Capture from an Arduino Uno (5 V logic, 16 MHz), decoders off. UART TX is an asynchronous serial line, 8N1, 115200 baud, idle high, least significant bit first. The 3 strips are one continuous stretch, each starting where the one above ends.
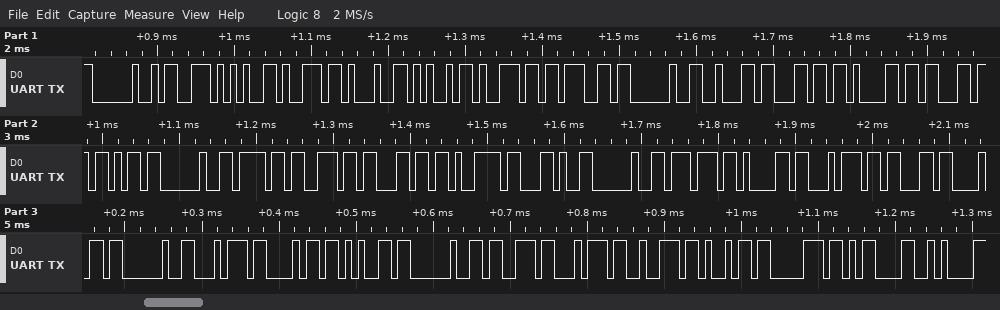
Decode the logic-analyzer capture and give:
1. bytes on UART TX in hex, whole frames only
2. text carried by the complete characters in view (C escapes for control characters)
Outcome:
20 73 65 6E 64 69 6E 67 20 62 6C 61 63 6B 20 6F 6E 6C 79 2C 20 77 61 74 63 68 20 74 68 65 20 73 74 72 69 70 0D 0A
" sending black only, watch the strip\r\n"
